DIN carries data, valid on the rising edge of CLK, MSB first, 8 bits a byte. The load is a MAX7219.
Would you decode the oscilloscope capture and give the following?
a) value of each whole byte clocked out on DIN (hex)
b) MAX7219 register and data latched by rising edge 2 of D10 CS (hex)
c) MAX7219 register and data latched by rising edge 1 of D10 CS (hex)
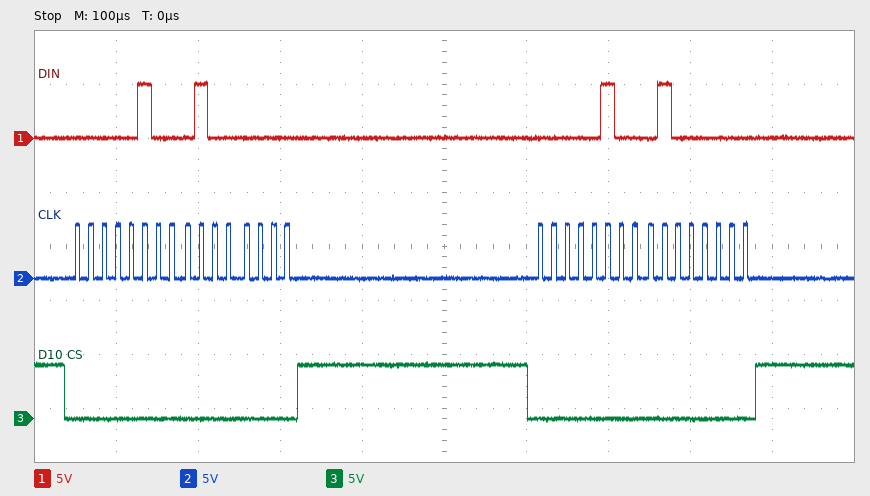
04 40 04 40
register 0x4, data 0x40
register 0x4, data 0x40
